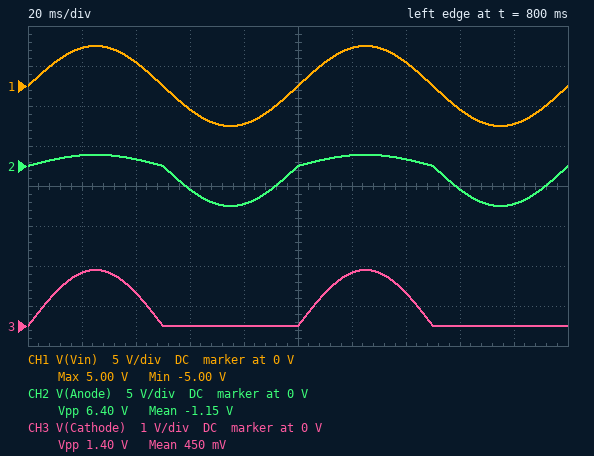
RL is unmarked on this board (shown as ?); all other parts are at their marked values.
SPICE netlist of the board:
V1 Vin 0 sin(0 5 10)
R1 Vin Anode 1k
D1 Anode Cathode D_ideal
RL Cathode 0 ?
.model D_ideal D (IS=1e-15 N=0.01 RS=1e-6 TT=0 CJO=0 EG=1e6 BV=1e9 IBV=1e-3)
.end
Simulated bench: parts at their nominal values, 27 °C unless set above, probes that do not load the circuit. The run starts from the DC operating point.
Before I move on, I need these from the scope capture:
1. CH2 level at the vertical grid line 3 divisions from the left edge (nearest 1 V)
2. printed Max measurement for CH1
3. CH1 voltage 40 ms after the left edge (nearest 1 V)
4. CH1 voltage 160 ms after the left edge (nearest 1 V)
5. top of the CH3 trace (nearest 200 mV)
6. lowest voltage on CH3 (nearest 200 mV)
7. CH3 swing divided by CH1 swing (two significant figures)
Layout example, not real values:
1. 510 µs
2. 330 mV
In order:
1. -3 V
2. 5.00 V
3. 3 V
4. -3 V
5. 1.4 V
6. 0 V
7. 0.14
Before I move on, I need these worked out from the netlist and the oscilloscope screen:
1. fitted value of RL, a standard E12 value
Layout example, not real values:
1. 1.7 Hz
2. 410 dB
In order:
1. 390 Ω
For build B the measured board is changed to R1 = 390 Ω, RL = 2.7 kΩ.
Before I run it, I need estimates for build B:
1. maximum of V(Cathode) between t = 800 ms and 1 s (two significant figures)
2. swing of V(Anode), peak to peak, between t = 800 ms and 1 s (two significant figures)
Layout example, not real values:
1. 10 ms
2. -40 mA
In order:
1. 4.4 V
2. 9.4 V
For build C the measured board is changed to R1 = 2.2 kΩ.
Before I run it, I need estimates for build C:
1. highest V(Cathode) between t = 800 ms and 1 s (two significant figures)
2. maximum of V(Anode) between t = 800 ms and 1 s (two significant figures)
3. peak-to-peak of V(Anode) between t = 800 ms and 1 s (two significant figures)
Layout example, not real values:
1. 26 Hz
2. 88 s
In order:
1. 750 mV
2. 760 mV
3. 5.8 V
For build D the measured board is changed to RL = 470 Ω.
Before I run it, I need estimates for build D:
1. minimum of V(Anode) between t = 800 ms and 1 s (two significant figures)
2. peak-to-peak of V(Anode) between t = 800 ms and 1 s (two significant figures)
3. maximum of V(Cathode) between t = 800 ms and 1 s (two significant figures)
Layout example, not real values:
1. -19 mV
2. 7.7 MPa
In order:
1. -5.0 V
2. 6.6 V
3. 1.6 V
